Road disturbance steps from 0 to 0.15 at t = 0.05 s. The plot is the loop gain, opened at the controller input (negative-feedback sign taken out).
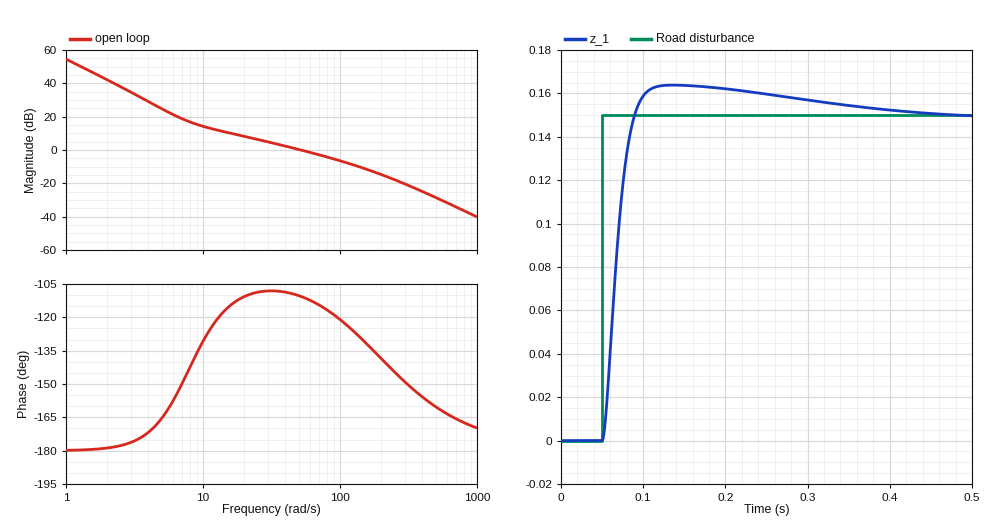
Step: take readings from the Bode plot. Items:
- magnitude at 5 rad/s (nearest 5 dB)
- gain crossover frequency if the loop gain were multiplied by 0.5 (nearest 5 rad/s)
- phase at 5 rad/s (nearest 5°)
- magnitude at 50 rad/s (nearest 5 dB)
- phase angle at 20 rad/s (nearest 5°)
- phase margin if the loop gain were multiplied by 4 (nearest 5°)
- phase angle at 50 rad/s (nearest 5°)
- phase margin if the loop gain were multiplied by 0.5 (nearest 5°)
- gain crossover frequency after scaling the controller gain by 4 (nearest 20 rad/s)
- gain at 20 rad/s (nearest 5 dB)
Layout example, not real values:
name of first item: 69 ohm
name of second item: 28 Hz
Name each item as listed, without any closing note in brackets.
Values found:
magnitude at 5 rad/s: 25 dB
gain crossover frequency if the loop gain were multiplied by 0.5: 25 rad/s
phase at 5 rad/s: -165°
magnitude at 50 rad/s: 0 dB
phase angle at 20 rad/s: -110°
phase margin if the loop gain were multiplied by 4: 45°
phase angle at 50 rad/s: -110°
phase margin if the loop gain were multiplied by 0.5: 70°
gain crossover frequency after scaling the controller gain by 4: 160 rad/s
gain at 20 rad/s: 10 dB
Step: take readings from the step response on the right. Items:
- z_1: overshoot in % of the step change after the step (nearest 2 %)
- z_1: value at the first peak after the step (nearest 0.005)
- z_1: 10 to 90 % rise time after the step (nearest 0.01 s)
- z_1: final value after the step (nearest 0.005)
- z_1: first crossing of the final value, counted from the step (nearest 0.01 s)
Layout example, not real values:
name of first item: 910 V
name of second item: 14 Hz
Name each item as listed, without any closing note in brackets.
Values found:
z_1: overshoot in % of the step change after the step: 10 %
z_1: value at the first peak after the step: 0.165
z_1: 10 to 90 % rise time after the step: 0.03 s
z_1: final value after the step: 0.150
z_1: first crossing of the final value, counted from the step: 0.04 s
